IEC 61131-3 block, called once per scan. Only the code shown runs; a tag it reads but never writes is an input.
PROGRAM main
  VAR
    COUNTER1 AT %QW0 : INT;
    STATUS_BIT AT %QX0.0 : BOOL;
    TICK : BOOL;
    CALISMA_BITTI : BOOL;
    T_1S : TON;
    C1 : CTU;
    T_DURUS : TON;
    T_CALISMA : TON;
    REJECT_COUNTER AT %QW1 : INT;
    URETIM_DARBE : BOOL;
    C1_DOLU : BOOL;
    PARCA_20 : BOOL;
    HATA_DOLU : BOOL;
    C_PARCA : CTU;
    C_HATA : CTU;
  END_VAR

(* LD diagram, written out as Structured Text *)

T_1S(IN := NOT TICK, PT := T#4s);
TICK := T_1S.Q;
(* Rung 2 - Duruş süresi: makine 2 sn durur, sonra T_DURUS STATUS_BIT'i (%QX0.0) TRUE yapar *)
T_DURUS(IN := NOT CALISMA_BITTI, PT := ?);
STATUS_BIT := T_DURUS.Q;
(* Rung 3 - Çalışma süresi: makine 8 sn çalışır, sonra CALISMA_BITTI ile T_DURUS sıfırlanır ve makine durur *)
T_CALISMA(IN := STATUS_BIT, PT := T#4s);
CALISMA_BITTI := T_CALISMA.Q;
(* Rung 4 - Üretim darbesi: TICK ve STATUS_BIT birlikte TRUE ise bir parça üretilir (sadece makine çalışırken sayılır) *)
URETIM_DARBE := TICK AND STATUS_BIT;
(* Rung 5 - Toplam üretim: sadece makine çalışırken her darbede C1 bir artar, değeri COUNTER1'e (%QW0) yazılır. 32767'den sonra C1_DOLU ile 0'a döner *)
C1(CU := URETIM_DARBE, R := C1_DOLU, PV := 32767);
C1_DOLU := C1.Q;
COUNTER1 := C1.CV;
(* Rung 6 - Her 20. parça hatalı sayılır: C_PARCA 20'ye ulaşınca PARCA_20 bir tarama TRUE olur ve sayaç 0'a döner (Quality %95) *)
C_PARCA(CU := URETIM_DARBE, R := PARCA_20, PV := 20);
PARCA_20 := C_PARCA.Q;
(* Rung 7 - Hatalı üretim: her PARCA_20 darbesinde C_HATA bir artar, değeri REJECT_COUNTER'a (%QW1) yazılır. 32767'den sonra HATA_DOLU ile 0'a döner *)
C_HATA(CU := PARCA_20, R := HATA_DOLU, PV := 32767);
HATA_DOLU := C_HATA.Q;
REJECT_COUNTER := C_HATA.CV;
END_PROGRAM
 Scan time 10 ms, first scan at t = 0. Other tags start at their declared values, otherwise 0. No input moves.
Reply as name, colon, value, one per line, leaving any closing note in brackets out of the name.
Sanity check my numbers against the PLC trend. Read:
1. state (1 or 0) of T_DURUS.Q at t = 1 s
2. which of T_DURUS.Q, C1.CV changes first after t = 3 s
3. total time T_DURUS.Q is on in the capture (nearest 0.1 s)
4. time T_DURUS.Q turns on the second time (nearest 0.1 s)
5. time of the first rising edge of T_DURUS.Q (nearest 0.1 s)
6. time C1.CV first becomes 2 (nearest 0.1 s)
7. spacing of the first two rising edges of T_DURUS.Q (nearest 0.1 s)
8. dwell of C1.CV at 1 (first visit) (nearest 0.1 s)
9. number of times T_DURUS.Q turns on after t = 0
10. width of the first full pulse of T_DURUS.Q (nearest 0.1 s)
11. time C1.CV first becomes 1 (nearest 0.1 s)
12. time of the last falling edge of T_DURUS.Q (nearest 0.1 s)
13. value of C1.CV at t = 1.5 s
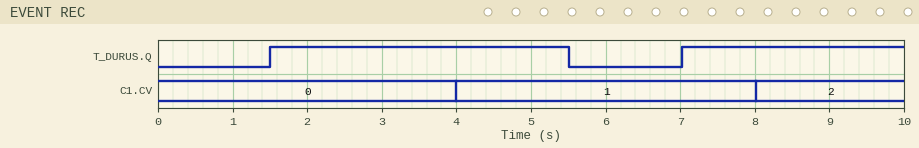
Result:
state (1 or 0) of T_DURUS.Q at t = 1 s: 0
which of T_DURUS.Q, C1.CV changes first after t = 3 s: C1.CV
total time T_DURUS.Q is on in the capture: 7.0 s
time T_DURUS.Q turns on the second time: 7.0 s
time of the first rising edge of T_DURUS.Q: 1.5 s
time C1.CV first becomes 2: 8.0 s
spacing of the first two rising edges of T_DURUS.Q: 5.5 s
dwell of C1.CV at 1 (first visit): 4.0 s
number of times T_DURUS.Q turns on after t = 0: 2
width of the first full pulse of T_DURUS.Q: 4.0 s
time C1.CV first becomes 1: 4.0 s
time of the last falling edge of T_DURUS.Q: 5.5 s
value of C1.CV at t = 1.5 s: 0
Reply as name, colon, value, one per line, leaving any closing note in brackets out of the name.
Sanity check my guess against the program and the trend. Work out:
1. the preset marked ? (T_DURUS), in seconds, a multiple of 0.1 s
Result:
the preset marked ? (T_DURUS), in seconds, a multiple of 0.1 s: 1.5 s
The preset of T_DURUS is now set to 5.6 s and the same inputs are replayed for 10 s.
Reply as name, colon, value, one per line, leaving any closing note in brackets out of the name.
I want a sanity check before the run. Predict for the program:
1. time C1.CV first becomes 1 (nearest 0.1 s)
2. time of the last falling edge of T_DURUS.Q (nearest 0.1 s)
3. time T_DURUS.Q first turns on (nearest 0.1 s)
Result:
time C1.CV first becomes 1: 8.0 s
time of the last falling edge of T_DURUS.Q: 9.6 s
time T_DURUS.Q first turns on: 5.6 s
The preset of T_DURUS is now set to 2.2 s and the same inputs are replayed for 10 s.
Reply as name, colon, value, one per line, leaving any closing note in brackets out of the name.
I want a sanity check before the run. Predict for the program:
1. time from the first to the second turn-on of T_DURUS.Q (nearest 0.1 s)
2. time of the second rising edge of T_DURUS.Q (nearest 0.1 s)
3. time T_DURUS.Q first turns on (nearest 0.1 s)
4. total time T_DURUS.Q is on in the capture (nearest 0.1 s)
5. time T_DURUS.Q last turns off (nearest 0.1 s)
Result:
time from the first to the second turn-on of T_DURUS.Q: 6.2 s
time of the second rising edge of T_DURUS.Q: 8.4 s
time T_DURUS.Q first turns on: 2.2 s
total time T_DURUS.Q is on in the capture: 5.6 s
time T_DURUS.Q last turns off: 6.2 s
